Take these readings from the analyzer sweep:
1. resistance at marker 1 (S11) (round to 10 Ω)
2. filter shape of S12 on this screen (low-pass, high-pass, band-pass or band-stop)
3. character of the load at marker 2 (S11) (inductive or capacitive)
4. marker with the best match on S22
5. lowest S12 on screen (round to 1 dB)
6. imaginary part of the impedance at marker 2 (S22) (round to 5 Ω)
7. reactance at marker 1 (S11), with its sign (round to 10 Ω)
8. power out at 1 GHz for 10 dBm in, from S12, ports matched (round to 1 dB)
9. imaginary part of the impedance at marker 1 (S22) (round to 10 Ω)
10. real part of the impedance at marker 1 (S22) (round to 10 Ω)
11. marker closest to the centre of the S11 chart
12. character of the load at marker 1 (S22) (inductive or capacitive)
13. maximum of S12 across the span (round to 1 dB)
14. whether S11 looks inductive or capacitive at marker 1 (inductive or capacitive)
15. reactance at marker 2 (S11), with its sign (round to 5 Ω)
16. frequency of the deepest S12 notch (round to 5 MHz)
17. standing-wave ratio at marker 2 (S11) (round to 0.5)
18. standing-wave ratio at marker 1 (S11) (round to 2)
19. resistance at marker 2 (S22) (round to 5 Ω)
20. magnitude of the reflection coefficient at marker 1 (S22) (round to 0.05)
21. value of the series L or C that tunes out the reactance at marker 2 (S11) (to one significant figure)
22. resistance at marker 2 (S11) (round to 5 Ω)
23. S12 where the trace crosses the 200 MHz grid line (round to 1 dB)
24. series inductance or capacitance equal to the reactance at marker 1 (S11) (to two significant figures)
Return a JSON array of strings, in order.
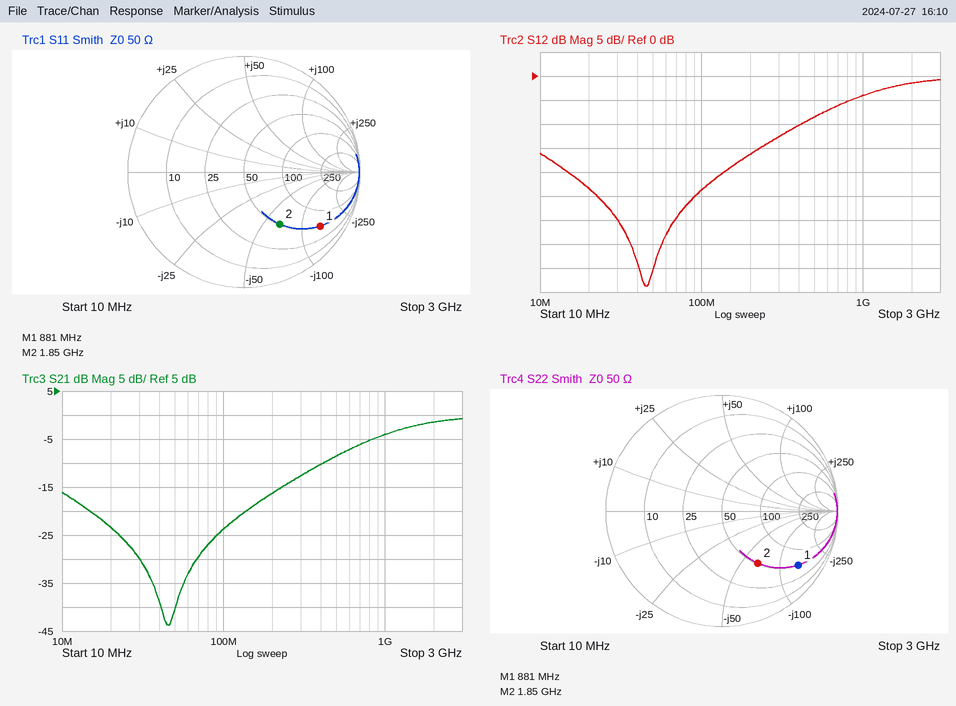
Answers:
["50 Ω", "high-pass", "capacitive", "marker 2", "-44 dB", "-65 Ω", "-140 Ω", "6 dBm", "-140 Ω", "50 Ω", "marker 2", "capacitive", "-1 dB", "capacitive", "-65 Ω", "45 MHz", "3.5", "10", "50 Ω", "0.80", "6 nH", "50 Ω", "-16 dB", "1.3 pF"]
